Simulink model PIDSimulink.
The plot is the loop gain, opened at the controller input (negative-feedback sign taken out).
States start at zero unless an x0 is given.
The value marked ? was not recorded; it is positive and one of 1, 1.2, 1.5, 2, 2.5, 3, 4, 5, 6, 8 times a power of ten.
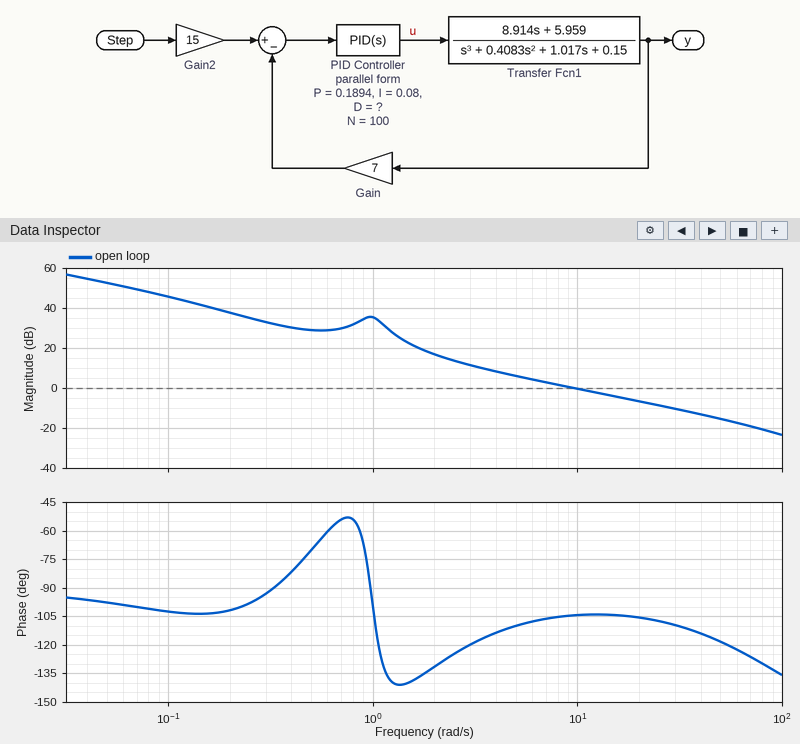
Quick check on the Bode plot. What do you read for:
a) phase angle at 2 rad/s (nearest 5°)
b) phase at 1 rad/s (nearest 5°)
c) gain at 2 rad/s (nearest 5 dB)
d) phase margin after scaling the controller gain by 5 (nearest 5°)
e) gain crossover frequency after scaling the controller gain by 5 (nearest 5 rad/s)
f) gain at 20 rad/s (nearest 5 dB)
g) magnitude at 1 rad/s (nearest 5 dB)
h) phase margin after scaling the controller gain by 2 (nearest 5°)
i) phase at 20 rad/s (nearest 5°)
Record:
-130°
-100°
15 dB
65°
45 rad/s
-5 dB
35 dB
75°
-105°
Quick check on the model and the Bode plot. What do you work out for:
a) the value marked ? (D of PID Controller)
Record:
0.15
